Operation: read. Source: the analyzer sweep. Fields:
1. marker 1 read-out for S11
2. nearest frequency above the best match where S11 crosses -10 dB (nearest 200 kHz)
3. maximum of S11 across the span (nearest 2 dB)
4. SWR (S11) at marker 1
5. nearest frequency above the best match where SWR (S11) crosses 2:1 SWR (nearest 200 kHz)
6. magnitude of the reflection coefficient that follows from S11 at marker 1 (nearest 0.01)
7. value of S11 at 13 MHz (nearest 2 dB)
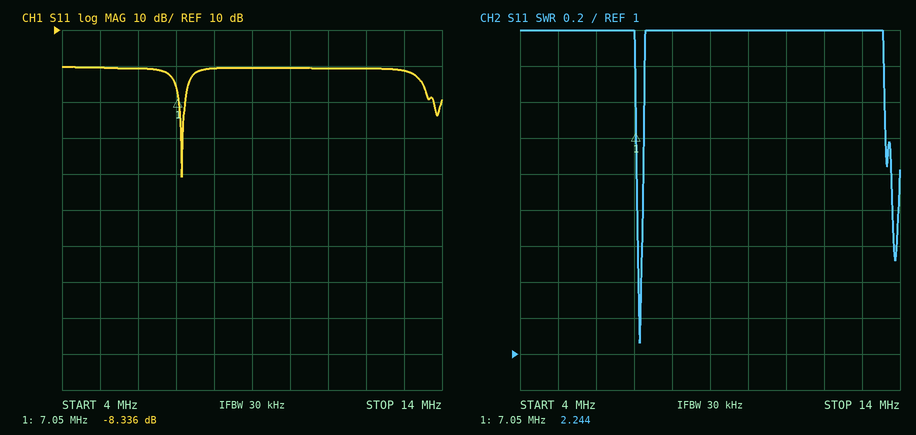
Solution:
-8.336 dB
7.2 MHz
0 dB
2.244
7.2 MHz
0.38
-2 dB
